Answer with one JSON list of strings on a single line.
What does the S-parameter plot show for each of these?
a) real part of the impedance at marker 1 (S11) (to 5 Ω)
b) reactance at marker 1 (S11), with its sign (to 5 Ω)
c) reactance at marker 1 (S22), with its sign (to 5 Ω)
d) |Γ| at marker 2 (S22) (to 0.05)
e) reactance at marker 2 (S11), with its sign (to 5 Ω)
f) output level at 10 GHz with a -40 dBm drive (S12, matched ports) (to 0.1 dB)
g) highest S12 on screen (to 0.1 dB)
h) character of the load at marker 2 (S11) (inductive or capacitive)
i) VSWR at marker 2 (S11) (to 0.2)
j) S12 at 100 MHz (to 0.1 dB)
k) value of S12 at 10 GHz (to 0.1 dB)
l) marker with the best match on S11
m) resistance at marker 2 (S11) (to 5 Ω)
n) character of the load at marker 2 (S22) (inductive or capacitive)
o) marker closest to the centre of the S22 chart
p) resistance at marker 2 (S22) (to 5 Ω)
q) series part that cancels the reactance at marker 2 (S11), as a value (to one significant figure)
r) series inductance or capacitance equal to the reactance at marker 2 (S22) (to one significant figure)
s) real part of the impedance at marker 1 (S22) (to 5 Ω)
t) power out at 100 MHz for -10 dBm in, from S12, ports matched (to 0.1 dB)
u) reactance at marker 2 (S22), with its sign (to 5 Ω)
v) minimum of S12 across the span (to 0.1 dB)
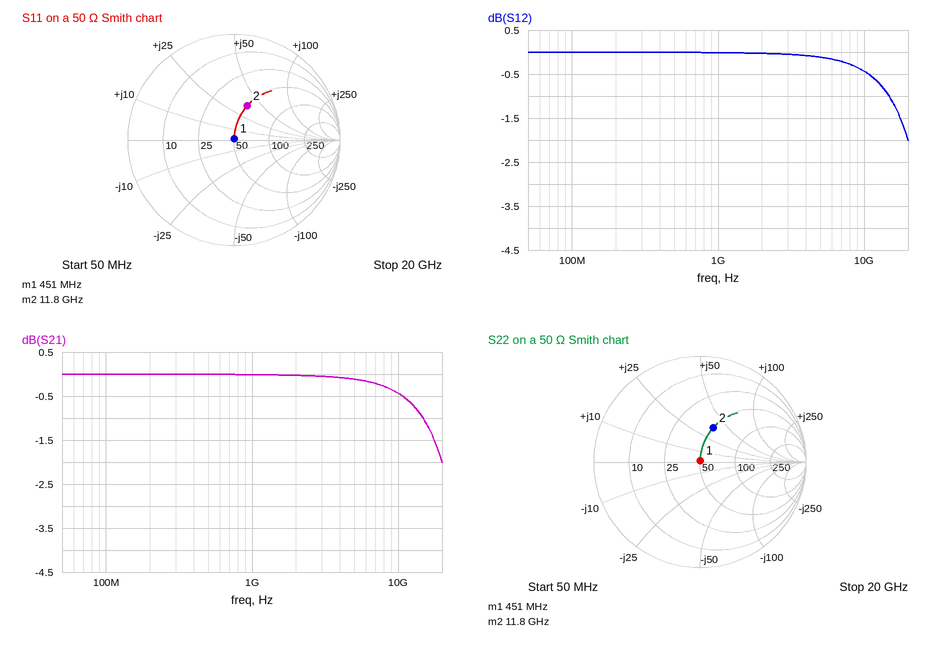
["50 Ω", "0 Ω", "0 Ω", "0.35", "+35 Ω", "-40.4 dBm", "0.0 dB", "inductive", "2.0", "0.0 dB", "-0.4 dB", "marker 1", "50 Ω", "inductive", "marker 1", "50 Ω", "400 fF", "500 pH", "50 Ω", "-10.0 dBm", "+35 Ω", "-2.0 dB"]
